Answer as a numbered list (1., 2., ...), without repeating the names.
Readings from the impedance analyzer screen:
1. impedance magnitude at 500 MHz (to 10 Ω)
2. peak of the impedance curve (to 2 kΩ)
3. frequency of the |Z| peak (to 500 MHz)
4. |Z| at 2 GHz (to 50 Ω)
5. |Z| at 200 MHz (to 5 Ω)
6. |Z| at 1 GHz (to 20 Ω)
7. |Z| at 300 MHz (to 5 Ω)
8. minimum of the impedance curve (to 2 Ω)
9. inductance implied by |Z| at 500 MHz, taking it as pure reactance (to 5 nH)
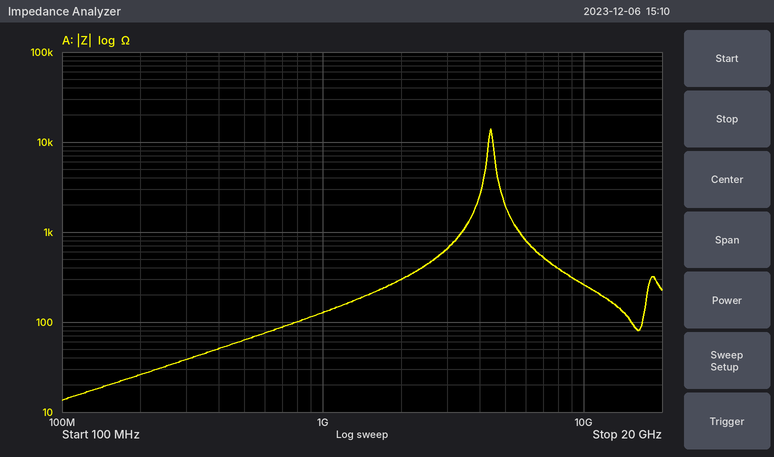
1. 60 Ω
2. 14 kΩ
3. 4.5 GHz
4. 300 Ω
5. 25 Ω
6. 120 Ω
7. 40 Ω
8. 14 Ω
9. 20 nH
